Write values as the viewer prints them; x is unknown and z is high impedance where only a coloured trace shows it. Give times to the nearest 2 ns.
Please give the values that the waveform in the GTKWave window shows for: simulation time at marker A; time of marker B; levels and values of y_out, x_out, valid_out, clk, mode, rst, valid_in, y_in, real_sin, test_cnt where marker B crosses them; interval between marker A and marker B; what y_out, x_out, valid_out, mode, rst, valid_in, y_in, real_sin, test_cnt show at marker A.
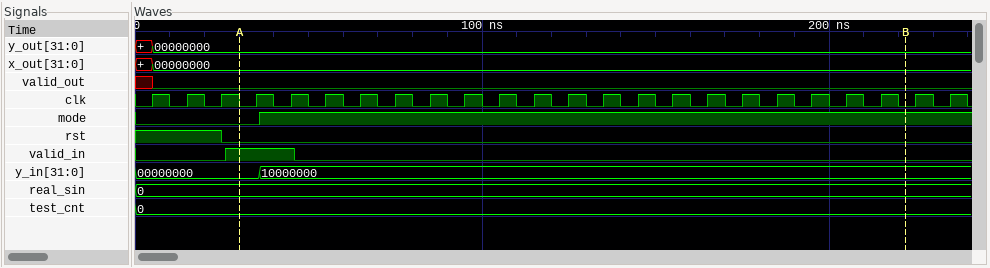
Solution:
30 ns
222 ns
y_out=00000000, x_out=00000000, valid_out=0, clk=0, mode=1, rst=0, valid_in=0, y_in=10000000, real_sin=0, test_cnt=0
192 ns
y_out=00000000, x_out=00000000, valid_out=0, mode=0, rst=0, valid_in=1, y_in=00000000, real_sin=0, test_cnt=0
